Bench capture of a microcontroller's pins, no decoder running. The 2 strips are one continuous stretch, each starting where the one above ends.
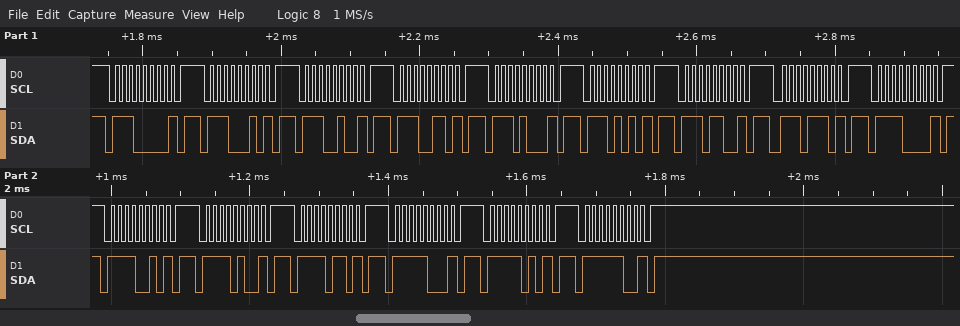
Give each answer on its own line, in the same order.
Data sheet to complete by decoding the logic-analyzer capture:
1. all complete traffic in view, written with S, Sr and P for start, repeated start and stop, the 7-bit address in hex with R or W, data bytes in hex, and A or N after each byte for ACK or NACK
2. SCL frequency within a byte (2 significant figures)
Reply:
S 70W N P S 71W N P S 72W N P S 73W N P S 74W N P S 75W N P S 76W N P S 77W N P S 78W N P S 79W N P S 7AW N P S 7BW N P S 7CW N P S 7DW N P S 7EW N P
100 kHz
